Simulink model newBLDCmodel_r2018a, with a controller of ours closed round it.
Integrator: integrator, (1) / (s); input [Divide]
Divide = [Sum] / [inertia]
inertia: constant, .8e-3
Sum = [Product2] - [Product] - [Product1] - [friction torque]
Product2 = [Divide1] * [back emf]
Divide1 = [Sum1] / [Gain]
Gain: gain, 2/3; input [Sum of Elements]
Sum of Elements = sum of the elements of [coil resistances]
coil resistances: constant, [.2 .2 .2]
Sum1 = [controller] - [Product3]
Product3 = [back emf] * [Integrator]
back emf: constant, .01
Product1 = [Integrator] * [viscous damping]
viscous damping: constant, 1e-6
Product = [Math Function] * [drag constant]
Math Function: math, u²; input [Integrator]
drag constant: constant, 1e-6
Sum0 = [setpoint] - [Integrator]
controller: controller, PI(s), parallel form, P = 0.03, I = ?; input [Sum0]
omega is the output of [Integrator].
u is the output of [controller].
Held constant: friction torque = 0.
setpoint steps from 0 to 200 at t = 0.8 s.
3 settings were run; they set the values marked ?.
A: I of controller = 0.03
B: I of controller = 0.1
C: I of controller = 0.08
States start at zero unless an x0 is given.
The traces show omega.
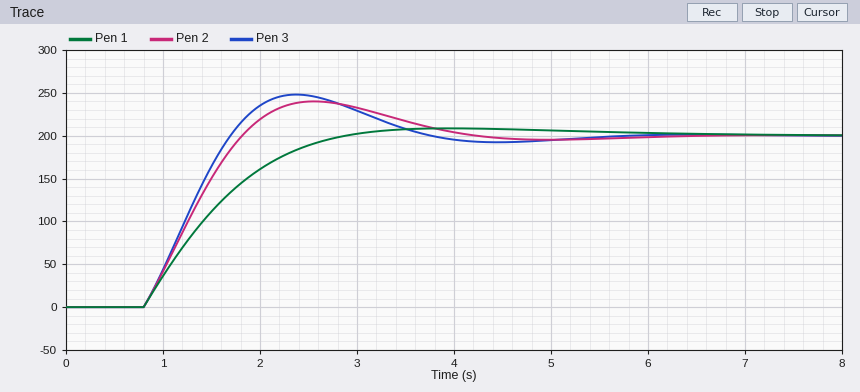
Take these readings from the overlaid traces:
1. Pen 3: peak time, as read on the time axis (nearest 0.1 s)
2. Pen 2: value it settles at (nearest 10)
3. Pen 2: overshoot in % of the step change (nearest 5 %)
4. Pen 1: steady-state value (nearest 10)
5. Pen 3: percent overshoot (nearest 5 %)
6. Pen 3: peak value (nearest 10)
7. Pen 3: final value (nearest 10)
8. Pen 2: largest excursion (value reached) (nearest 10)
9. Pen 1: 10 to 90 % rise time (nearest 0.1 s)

2.4 s
200
20 %
200
25 %
250
200
240
1.4 s
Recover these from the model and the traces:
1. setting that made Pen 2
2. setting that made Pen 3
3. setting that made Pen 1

C
B
A
